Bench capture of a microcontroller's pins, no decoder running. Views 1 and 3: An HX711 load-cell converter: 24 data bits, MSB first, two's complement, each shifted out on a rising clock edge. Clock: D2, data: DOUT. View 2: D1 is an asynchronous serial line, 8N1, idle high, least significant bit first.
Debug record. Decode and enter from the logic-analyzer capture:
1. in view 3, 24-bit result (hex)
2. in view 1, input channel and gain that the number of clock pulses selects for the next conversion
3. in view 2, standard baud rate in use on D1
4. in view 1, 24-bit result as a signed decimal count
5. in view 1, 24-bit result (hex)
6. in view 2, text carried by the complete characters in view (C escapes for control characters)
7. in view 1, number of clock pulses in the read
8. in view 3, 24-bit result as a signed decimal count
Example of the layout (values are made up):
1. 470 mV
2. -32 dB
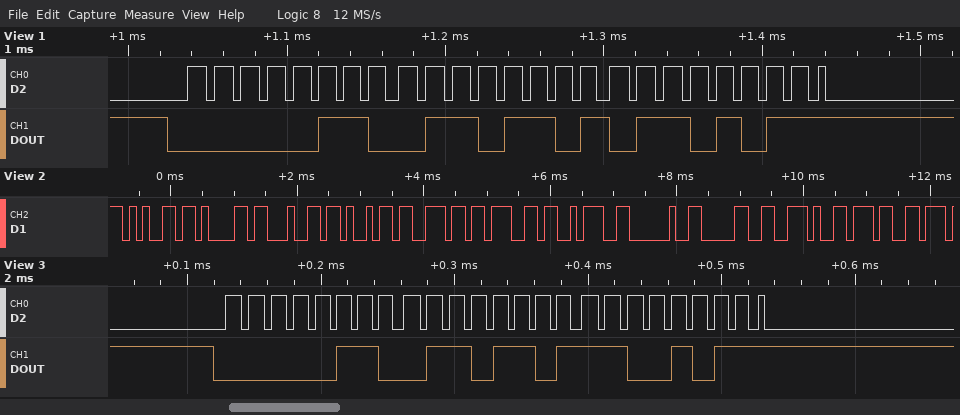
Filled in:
1. 0x066DCB
2. channel A, gain 128
3. 9600 baud
4. 421227
5. 0x066D6B
6. "eading: 0.7"
7. 25
8. 421323
